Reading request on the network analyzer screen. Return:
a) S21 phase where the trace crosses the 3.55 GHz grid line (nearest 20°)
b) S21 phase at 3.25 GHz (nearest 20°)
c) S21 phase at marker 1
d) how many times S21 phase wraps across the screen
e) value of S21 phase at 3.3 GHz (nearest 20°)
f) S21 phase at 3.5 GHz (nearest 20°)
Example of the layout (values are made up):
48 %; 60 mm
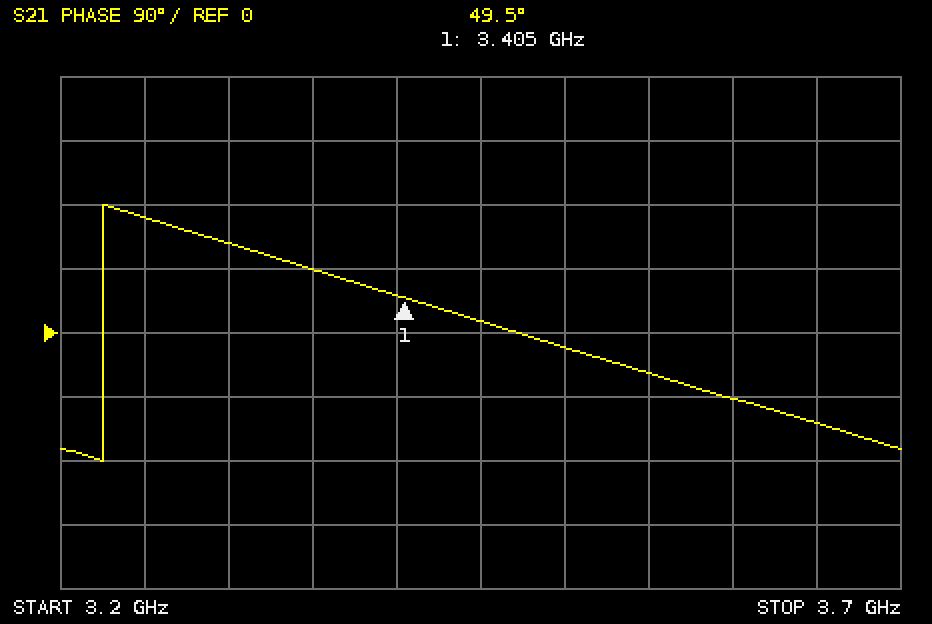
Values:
-60°; 160°; 49.5°; 1; 120°; -20°
